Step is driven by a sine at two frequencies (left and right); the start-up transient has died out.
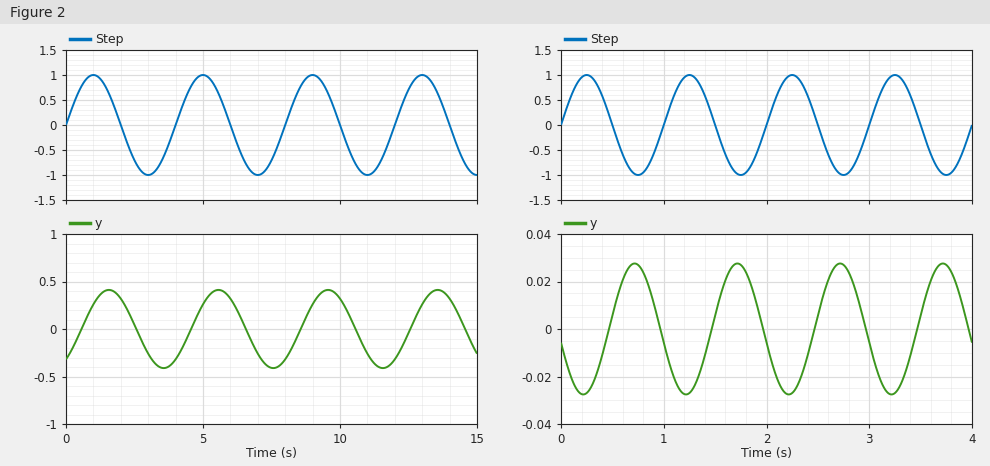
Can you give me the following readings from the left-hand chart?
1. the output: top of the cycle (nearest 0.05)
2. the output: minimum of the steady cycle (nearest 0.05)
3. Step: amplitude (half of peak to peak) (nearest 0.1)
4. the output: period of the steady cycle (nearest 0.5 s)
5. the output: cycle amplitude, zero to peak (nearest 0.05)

0.40
-0.40
1.0
4.0 s
0.40
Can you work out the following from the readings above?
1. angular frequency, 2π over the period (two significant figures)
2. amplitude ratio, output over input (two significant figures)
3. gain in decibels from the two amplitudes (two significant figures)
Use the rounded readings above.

1.6 rad/s
0.40
-8.0 dB
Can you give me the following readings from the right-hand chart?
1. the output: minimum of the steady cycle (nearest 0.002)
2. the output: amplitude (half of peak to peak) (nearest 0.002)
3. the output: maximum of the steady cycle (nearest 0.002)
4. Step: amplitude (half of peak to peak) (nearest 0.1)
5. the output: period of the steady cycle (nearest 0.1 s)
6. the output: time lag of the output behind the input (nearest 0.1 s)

-0.028
0.028
0.028
1.0
1.0 s
0.5 s
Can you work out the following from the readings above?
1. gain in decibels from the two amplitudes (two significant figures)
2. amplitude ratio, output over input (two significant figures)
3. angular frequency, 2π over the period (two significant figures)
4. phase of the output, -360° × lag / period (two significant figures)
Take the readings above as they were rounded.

-31 dB
0.028
6.3 rad/s
-180°
